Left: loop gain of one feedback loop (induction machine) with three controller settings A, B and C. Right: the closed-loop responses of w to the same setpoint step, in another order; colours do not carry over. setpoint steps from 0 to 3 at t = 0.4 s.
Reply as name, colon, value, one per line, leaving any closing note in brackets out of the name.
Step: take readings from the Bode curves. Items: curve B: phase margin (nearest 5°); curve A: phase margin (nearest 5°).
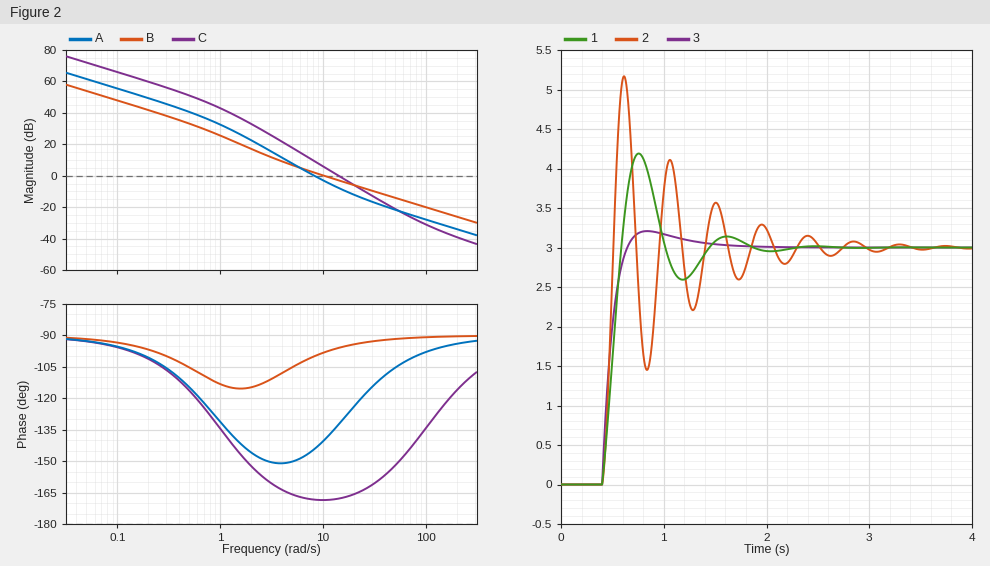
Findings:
curve B: phase margin: 80°
curve A: phase margin: 35°
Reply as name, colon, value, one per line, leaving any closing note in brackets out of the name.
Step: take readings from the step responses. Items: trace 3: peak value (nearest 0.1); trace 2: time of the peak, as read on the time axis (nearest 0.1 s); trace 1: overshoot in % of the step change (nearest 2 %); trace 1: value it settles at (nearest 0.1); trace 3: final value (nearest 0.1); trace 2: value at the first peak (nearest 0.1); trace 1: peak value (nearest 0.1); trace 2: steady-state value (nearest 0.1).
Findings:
trace 3: peak value: 3.2
trace 2: time of the peak, as read on the time axis: 0.6 s
trace 1: overshoot in % of the step change: 40 %
trace 1: value it settles at: 3.0
trace 3: final value: 3.0
trace 2: value at the first peak: 5.2
trace 1: peak value: 4.2
trace 2: steady-state value: 3.0
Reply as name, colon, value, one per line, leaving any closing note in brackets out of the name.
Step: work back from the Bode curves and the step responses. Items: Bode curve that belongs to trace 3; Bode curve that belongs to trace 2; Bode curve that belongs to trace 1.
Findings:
Bode curve that belongs to trace 3: B
Bode curve that belongs to trace 2: C
Bode curve that belongs to trace 1: A
